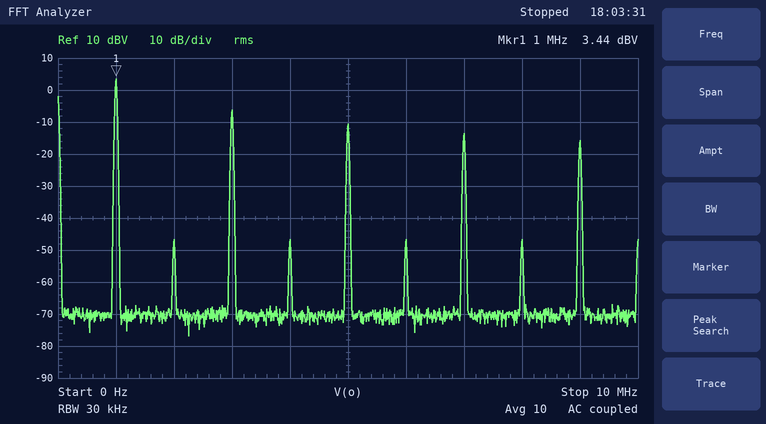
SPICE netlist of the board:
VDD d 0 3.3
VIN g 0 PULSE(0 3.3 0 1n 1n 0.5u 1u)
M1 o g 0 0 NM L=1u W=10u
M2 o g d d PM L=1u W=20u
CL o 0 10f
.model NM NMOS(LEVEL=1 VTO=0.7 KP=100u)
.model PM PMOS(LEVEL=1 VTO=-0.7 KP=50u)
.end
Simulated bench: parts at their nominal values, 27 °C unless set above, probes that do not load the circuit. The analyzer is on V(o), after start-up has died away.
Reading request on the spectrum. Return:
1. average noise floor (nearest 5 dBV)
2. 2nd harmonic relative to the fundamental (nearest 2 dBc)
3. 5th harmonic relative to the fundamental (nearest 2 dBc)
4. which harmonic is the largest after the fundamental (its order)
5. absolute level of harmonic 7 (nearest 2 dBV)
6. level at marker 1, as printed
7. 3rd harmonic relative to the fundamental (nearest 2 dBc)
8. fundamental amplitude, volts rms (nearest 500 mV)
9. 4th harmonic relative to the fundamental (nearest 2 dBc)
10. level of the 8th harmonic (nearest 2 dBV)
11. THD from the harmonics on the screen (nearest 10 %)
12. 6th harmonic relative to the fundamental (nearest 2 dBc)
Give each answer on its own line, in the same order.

-70 dBV
-50 dBc
-14 dBc
3
-14 dBV
3.44 dBV
-10 dBc
1.5 V
-50 dBc
-46 dBV
40 %
-50 dBc
